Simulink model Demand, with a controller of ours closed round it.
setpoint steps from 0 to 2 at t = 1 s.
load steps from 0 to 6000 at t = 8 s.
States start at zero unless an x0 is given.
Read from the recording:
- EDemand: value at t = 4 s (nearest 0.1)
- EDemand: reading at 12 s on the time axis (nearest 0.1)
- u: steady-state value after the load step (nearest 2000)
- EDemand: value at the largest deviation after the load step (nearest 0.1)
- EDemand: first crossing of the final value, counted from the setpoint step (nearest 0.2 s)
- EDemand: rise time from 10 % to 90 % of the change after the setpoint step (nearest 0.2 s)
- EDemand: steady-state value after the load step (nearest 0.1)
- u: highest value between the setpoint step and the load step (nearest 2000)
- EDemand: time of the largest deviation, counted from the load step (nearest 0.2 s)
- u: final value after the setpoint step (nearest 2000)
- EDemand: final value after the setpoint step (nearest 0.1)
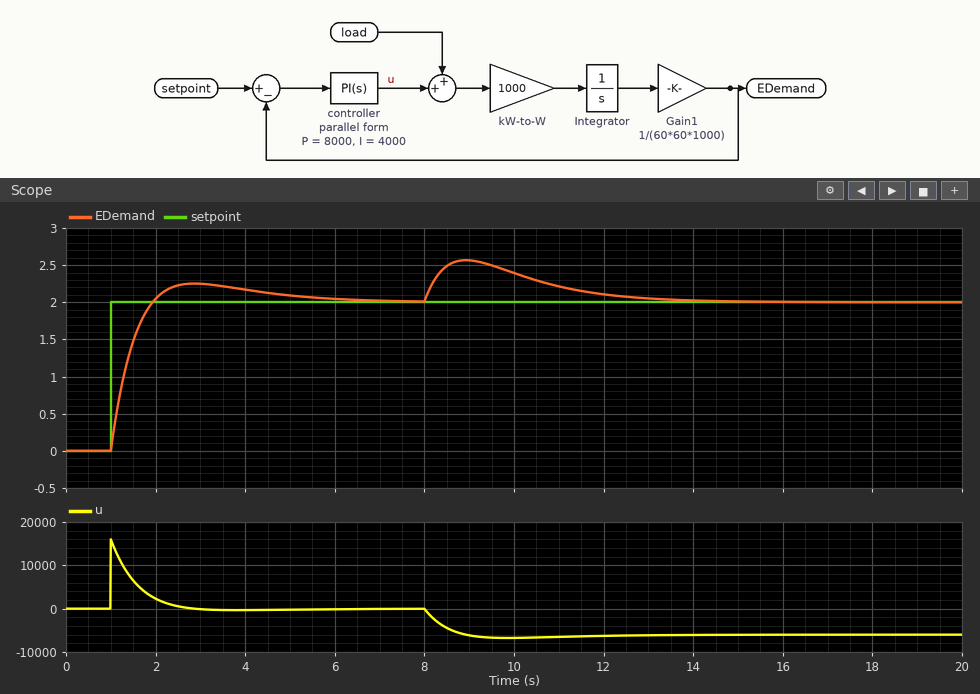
2.2
2.1
-6000
2.6
1.0 s
0.6 s
2.0
16000
1.0 s
0
2.0
